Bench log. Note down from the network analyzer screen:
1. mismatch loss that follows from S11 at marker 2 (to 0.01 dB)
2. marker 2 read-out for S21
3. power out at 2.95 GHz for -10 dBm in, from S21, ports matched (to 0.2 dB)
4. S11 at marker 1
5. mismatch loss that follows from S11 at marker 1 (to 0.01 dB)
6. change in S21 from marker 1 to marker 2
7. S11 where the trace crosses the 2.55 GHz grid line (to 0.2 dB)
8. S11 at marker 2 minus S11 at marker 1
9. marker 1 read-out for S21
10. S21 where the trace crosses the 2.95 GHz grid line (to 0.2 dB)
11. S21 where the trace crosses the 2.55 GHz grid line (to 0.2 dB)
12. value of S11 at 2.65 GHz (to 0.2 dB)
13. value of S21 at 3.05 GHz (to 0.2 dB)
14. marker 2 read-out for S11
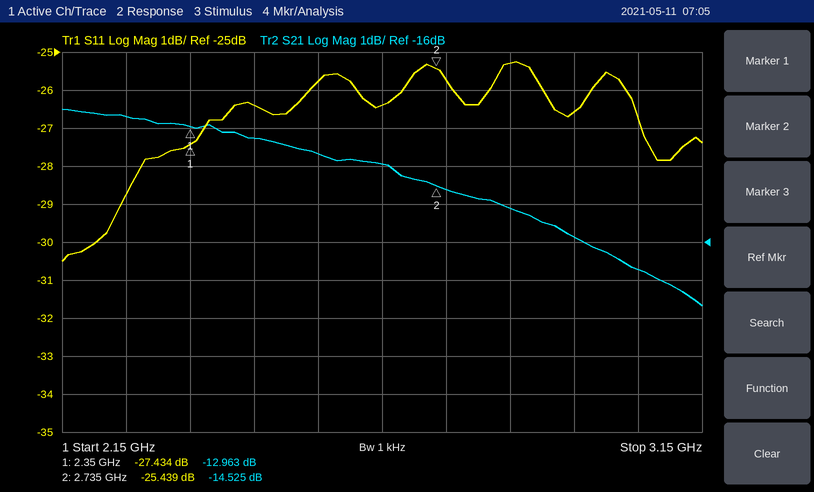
0.01 dB
-14.525 dB
-25.8 dBm
-27.434 dB
0.01 dB
-1.562 dB
-25.8 dB
1.995 dB
-12.963 dB
-15.8 dB
-13.6 dB
-26.4 dB
-16.8 dB
-25.439 dB
